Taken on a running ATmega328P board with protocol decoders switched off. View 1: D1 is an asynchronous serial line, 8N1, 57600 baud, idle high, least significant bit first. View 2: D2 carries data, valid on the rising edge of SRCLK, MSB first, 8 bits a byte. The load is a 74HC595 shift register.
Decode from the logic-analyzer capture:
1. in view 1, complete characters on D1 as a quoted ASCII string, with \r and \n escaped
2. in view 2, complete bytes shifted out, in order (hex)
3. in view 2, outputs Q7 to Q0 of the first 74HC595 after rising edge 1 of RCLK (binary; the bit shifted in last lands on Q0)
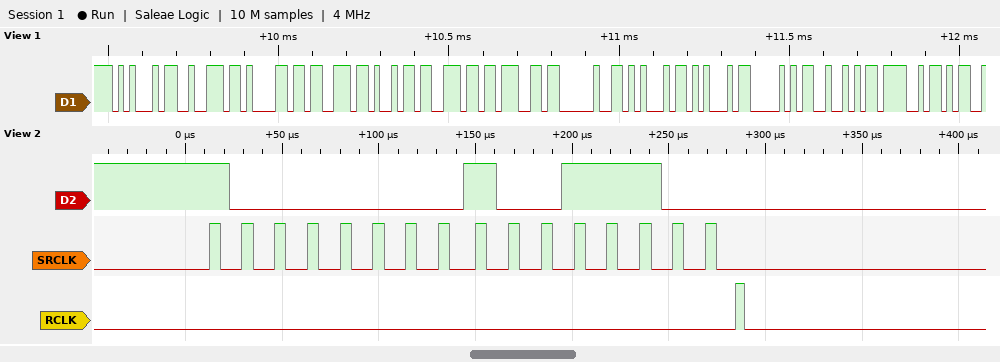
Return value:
"Erasing EEPRO"
0x80 0x9C
10011100
